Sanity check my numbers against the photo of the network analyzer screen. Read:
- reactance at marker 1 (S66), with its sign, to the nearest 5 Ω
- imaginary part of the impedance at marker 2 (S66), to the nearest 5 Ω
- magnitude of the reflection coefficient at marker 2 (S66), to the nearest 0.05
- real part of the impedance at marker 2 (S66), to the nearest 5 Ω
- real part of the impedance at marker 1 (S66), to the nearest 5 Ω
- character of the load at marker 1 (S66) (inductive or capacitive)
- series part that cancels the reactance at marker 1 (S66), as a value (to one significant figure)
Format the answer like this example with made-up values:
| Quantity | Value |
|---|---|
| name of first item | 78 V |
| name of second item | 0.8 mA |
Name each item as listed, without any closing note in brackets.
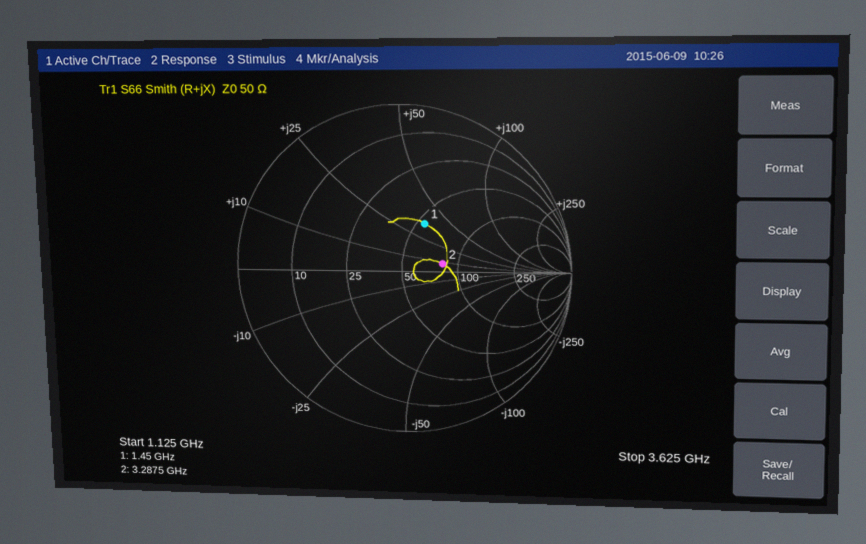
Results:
| Quantity | Value |
|---|---|
| reactance at marker 1 (S66), with its sign, to the nearest 5 Ω | +35 Ω |
| imaginary part of the impedance at marker 2 (S66), to the nearest 5 Ω | +10 Ω |
| magnitude of the reflection coefficient at marker 2 (S66), to the nearest 0.05 | 0.25 |
| real part of the impedance at marker 2 (S66), to the nearest 5 Ω | 80 Ω |
| real part of the impedance at marker 1 (S66), to the nearest 5 Ω | 55 Ω |
| character of the load at marker 1 (S66) | inductive |
| series part that cancels the reactance at marker 1 (S66), as a value | 3 pF |
